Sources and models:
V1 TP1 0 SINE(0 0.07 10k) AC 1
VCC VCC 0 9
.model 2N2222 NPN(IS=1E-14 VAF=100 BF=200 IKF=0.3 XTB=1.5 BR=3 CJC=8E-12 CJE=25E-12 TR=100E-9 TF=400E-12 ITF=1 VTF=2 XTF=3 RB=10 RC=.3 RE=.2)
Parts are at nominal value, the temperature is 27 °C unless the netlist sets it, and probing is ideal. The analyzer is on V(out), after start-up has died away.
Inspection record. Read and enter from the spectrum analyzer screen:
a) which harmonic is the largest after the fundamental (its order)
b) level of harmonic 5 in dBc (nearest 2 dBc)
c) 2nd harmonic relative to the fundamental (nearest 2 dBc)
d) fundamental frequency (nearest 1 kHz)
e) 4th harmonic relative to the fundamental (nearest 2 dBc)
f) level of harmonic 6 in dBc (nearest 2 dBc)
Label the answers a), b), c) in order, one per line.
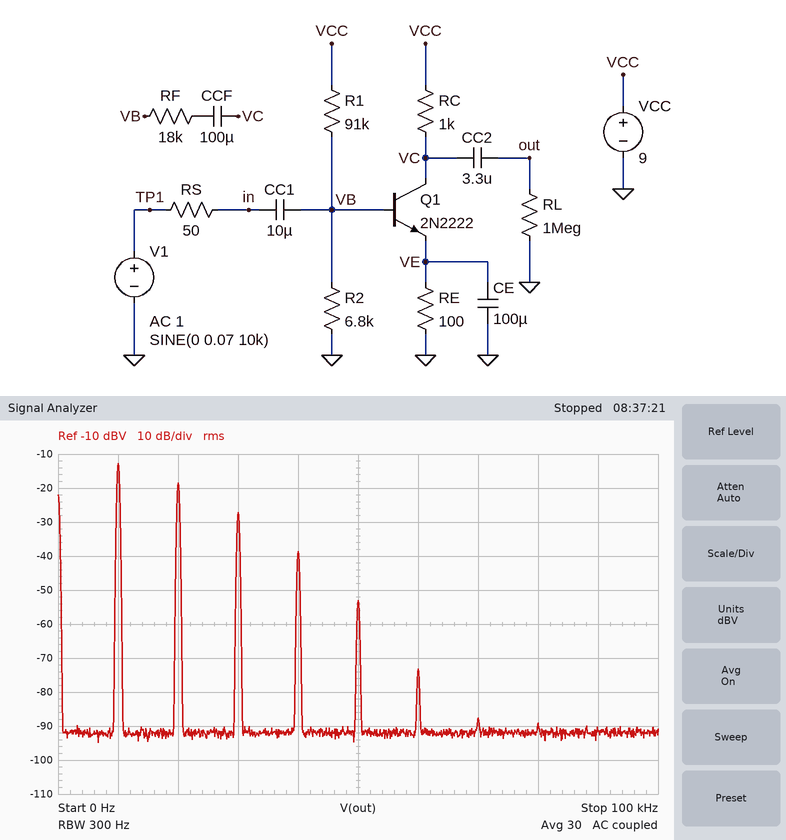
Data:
a) 2
b) -40 dBc
c) -6 dBc
d) 10 kHz
e) -26 dBc
f) -60 dBc
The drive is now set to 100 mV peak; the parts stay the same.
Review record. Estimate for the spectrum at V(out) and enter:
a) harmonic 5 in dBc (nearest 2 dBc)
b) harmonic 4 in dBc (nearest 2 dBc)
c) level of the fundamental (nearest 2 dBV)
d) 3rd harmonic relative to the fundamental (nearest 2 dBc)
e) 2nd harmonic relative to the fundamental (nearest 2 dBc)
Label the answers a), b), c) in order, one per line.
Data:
a) -30 dBc
b) -20 dBc
c) -10 dBV
d) -10 dBc
e) -4 dBc
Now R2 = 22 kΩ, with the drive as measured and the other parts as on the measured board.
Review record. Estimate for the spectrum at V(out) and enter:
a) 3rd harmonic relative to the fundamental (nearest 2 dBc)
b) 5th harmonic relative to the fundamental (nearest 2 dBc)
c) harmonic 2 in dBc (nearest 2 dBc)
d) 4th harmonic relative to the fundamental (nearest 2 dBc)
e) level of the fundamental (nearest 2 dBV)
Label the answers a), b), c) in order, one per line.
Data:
a) -16 dBc
b) -46 dBc
c) -22 dBc
d) -22 dBc
e) 10 dBV
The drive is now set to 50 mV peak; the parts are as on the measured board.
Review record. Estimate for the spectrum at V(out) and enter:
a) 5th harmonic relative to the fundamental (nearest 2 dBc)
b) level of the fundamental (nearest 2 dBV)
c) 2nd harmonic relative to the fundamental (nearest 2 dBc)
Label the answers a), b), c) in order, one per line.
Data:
a) -50 dBc
b) -16 dBV
c) -8 dBc
